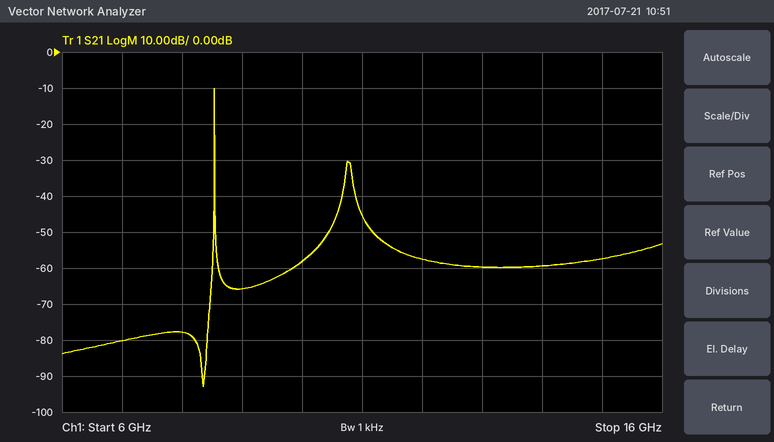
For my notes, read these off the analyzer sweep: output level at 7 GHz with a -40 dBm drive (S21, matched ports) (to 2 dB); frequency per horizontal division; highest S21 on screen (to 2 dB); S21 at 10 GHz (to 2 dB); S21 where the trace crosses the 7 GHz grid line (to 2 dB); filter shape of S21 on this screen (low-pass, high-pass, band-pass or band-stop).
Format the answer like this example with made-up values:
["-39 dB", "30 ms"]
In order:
["-120 dBm", "1 GHz", "-10 dB", "-58 dB", "-80 dB", "band-pass"]
